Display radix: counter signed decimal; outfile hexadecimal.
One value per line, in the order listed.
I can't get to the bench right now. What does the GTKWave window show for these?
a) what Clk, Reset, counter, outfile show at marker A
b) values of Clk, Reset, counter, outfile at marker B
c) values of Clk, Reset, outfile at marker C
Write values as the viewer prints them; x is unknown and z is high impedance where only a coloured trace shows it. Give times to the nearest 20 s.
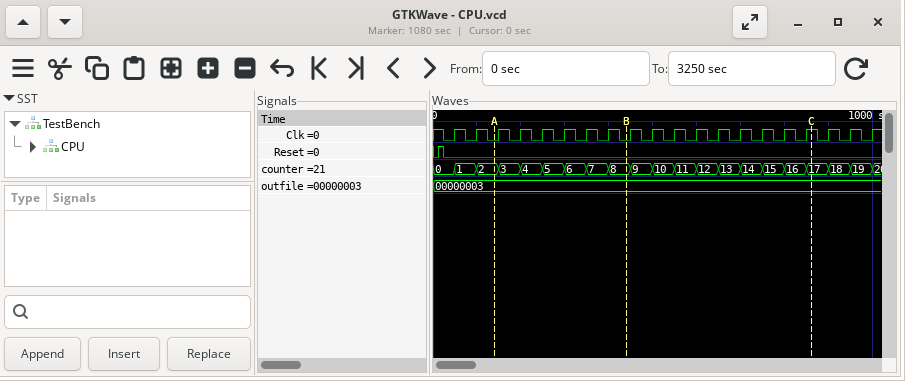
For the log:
Clk=0, Reset=0, counter=2, outfile=00000003
Clk=0, Reset=0, counter=8, outfile=00000003
Clk=1, Reset=0, outfile=00000003
